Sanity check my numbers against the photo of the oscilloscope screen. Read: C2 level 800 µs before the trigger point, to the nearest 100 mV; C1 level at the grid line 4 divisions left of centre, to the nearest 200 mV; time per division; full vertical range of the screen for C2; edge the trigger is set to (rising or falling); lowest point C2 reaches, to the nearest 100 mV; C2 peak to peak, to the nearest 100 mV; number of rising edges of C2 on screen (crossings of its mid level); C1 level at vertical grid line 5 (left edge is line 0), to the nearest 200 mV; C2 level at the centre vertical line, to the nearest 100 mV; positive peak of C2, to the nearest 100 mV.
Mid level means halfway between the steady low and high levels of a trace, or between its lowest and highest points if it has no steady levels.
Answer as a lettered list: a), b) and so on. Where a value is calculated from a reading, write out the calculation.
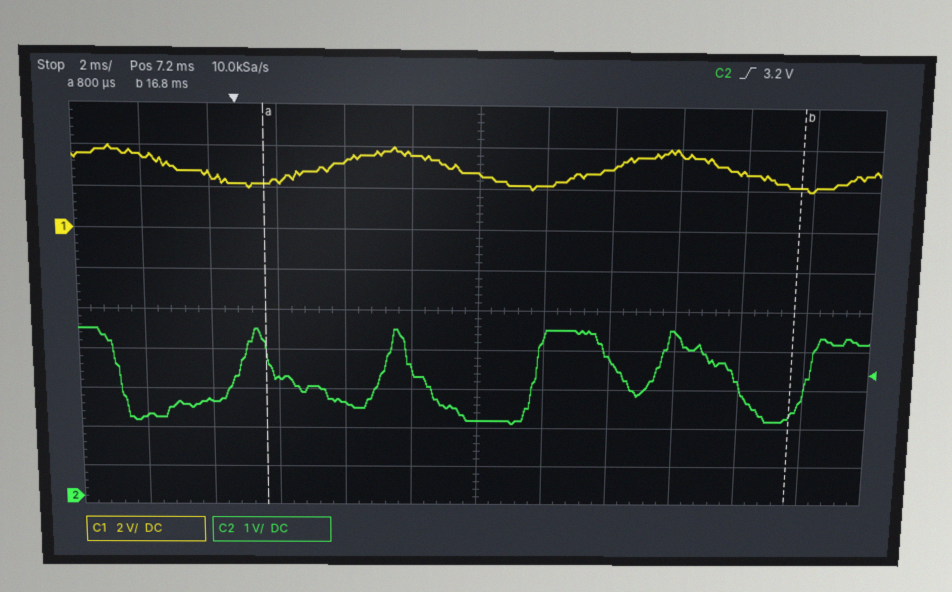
a) 2.5 V
b) 2.6 V
c) 2 ms
d) 10 V
e) rising
f) 1.9 V
g) 4.3 V − (1.9 V) = 2.4 V
h) 5
i) 3.6 V
j) 2.0 V
k) 4.3 V
